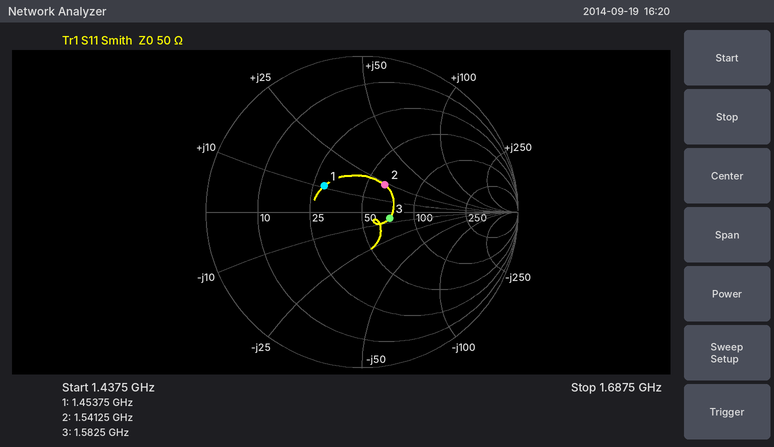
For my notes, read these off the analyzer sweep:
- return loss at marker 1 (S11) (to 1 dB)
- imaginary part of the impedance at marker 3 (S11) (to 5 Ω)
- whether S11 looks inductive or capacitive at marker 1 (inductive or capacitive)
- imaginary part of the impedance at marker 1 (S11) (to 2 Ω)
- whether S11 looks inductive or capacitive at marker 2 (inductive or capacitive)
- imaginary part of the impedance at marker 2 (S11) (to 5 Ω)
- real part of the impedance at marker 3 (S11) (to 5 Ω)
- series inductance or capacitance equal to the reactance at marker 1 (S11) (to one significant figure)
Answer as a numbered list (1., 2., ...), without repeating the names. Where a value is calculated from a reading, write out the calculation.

1. 11 dB
2. -5 Ω
3. inductive
4. +10 Ω
5. inductive
6. +25 Ω
7. 70 Ω
8. L = 10 Ω/(2π × 1.45375 GHz) ≈ 1 nH
